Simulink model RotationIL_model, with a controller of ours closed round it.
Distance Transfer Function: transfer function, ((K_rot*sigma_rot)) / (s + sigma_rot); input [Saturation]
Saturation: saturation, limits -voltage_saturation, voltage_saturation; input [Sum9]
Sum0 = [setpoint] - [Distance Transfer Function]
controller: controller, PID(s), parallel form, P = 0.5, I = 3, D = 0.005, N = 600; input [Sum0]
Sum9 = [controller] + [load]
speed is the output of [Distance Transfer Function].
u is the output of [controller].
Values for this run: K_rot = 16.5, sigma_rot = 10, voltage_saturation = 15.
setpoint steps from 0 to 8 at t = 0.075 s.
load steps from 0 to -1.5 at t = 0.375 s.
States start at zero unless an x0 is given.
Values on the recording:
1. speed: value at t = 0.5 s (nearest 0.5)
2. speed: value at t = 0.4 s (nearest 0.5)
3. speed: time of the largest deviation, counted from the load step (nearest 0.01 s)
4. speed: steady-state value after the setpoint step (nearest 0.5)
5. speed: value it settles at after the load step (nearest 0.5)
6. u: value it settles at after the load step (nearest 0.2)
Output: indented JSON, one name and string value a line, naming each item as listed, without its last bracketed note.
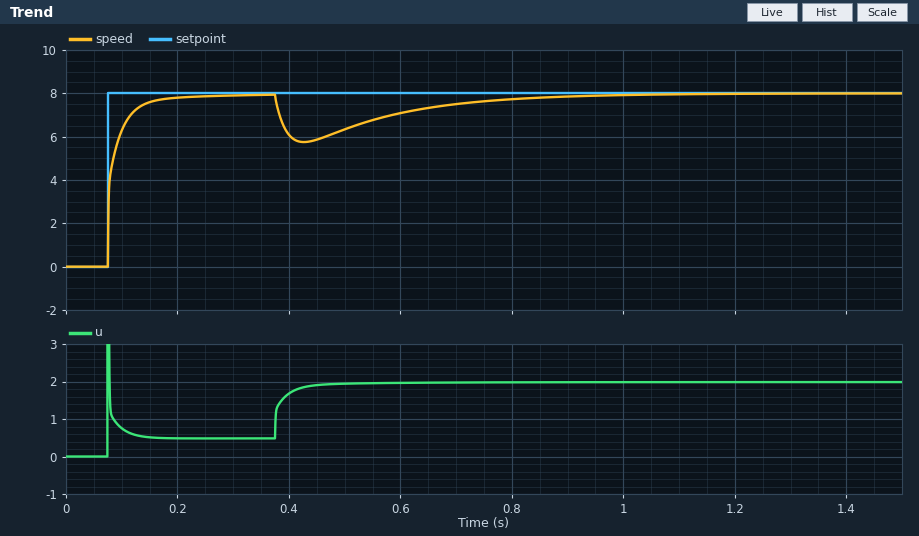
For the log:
{
  "speed: value at t = 0.5 s": "6.5",
  "speed: value at t = 0.4 s": "6.0",
  "speed: time of the largest deviation, counted from the load step": "0.05 s",
  "speed: steady-state value after the setpoint step": "8.0",
  "speed: value it settles at after the load step": "8.0",
  "u: value it settles at after the load step": "2.0"
}
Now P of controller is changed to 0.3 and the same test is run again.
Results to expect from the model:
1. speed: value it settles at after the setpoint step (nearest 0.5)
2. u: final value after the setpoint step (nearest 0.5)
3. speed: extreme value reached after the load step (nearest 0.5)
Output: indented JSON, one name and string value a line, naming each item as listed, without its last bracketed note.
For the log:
{
  "speed: value it settles at after the setpoint step": "8.0",
  "u: final value after the setpoint step": "0.5",
  "speed: extreme value reached after the load step": "5.0"
}
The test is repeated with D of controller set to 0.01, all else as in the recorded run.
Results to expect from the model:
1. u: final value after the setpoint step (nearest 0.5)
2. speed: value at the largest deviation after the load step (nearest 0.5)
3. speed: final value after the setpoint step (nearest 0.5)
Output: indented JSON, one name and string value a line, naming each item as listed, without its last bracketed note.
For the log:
{
  "u: final value after the setpoint step": "0.5",
  "speed: value at the largest deviation after the load step": "6.0",
  "speed: final value after the setpoint step": "8.0"
}
